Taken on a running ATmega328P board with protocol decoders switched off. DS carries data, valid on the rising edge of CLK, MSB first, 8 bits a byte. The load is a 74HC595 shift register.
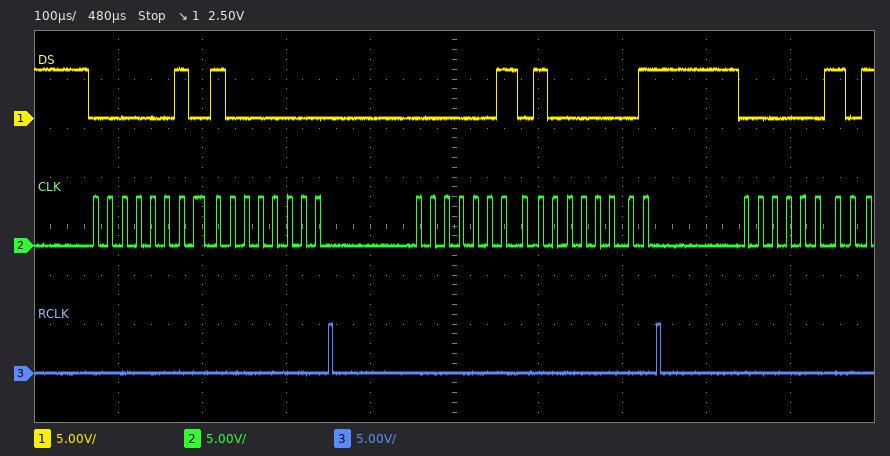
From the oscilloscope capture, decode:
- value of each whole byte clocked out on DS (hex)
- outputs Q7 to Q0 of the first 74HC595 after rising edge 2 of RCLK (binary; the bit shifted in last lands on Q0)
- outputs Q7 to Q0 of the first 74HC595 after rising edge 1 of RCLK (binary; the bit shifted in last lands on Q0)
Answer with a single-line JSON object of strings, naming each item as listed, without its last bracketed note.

{"value of each whole byte clocked out on DS": "02 80 02 81 02", "outputs Q7 to Q0 of the first 74HC595 after rising edge 2 of RCLK": "10000001", "outputs Q7 to Q0 of the first 74HC595 after rising edge 1 of RCLK": "10000000"}
